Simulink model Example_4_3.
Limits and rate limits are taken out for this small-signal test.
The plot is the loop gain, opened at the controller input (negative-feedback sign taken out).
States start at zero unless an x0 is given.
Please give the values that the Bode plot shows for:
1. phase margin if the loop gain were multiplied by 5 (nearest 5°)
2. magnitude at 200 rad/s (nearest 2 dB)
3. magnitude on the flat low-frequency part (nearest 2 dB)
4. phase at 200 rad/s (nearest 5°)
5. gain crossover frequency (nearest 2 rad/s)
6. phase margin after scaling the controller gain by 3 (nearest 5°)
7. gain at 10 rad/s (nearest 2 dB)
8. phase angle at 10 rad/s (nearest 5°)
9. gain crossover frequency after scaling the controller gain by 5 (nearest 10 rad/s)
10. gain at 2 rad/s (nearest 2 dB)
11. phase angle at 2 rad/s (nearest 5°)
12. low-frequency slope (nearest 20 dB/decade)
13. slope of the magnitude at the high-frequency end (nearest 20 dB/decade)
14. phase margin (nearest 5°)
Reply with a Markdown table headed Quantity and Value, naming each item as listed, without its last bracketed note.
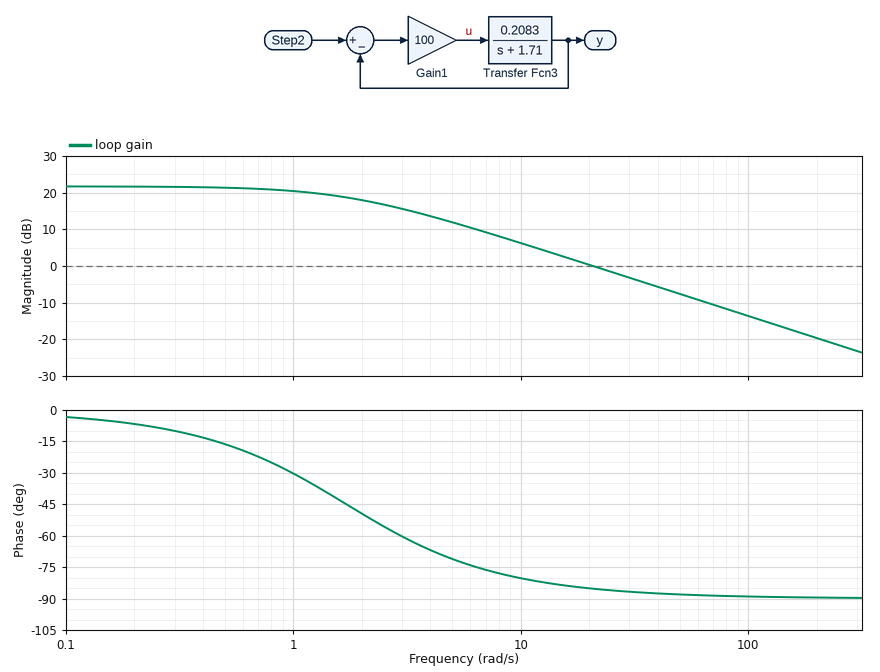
| Quantity | Value |
|---|---|
| phase margin if the loop gain were multiplied by 5 | 90° |
| magnitude at 200 rad/s | -20 dB |
| magnitude on the flat low-frequency part | 22 dB |
| phase at 200 rad/s | -90° |
| gain crossover frequency | 20 rad/s |
| phase margin after scaling the controller gain by 3 | 90° |
| gain at 10 rad/s | 6 dB |
| phase angle at 10 rad/s | -80° |
| gain crossover frequency after scaling the controller gain by 5 | 100 rad/s |
| gain at 2 rad/s | 18 dB |
| phase angle at 2 rad/s | -50° |
| low-frequency slope | 0 dB/decade |
| slope of the magnitude at the high-frequency end | -20 dB/decade |
| phase margin | 95° |
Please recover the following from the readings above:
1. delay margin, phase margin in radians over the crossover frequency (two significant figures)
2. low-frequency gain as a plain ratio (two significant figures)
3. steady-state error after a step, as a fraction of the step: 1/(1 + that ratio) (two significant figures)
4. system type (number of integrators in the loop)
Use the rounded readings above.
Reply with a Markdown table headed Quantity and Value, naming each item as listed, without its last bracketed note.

| Quantity | Value |
|---|---|
| delay margin, phase margin in radians over the crossover frequency | 0.083 s |
| low-frequency gain as a plain ratio | 13 |
| steady-state error after a step, as a fraction of the step: 1/(1 + that ratio) | 0.071 |
| system type | 0 |
